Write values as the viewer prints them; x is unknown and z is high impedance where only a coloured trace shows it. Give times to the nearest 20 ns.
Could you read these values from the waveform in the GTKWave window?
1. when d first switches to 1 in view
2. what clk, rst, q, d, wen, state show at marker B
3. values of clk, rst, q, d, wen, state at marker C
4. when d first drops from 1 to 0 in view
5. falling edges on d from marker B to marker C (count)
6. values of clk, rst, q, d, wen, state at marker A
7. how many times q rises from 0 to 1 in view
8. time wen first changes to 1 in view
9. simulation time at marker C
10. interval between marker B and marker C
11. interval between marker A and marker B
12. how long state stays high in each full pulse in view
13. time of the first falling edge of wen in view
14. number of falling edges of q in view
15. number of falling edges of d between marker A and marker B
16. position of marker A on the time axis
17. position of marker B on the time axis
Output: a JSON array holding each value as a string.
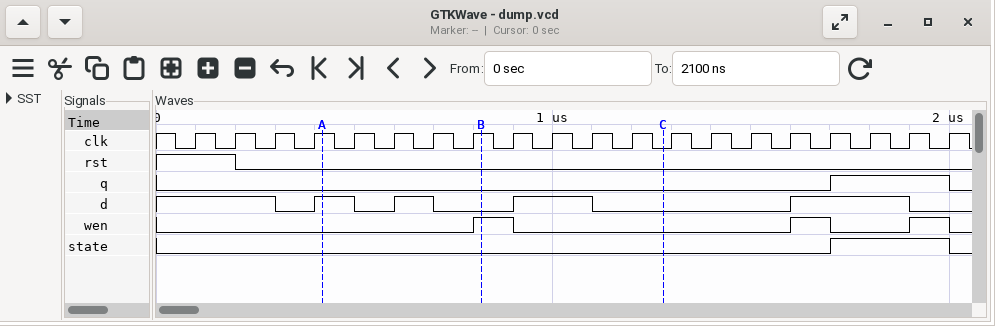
["400 ns", "clk=1, rst=0, q=0, d=0, wen=1, state=0", "clk=0, rst=0, q=0, d=0, wen=0, state=0", "300 ns", "1", "clk=1, rst=0, q=0, d=1, wen=0, state=0", "1", "800 ns", "1280 ns", "460 ns", "400 ns", "300 ns", "900 ns", "1", "2", "420 ns", "820 ns"]
